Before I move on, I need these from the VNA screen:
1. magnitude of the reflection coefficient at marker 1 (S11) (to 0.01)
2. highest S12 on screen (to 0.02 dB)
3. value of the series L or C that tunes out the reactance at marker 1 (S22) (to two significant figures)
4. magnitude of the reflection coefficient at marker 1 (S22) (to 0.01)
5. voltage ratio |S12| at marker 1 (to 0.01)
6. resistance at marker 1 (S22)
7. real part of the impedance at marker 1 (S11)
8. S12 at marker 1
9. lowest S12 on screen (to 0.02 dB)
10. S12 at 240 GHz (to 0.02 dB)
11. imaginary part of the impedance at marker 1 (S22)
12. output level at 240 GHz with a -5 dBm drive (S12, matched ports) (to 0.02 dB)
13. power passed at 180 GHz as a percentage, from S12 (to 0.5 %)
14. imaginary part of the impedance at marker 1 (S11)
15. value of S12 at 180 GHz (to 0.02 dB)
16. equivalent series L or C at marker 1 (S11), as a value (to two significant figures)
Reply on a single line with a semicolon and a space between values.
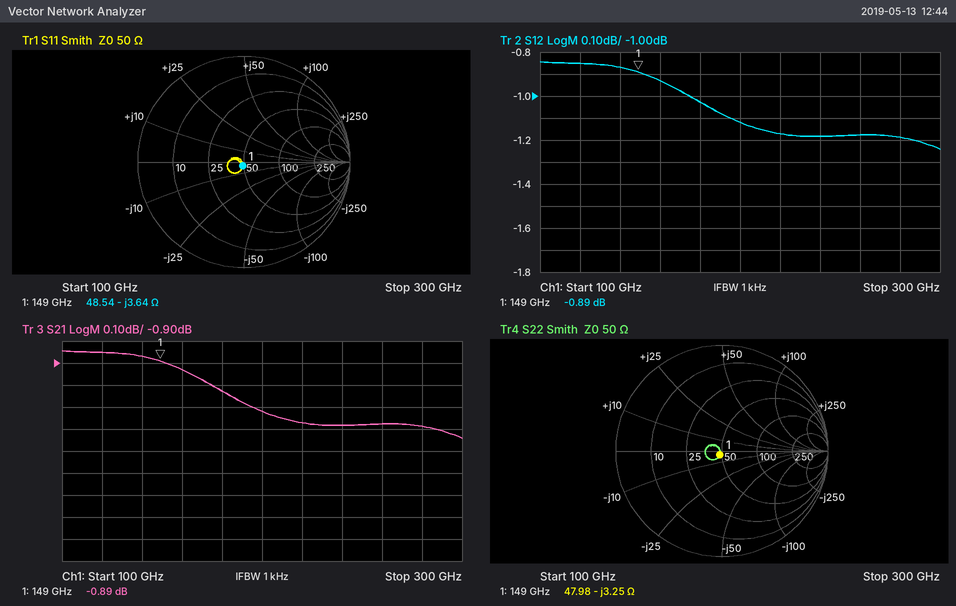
0.04; -0.84 dB; 3.5 pH; 0.04; 0.90; 47.98 Ω; 48.54 Ω; -0.89 dB; -1.24 dB; -1.18 dB; -3.25 Ω; -6.18 dBm; 79.0 %; -3.64 Ω; -1.02 dB; 290 fF
